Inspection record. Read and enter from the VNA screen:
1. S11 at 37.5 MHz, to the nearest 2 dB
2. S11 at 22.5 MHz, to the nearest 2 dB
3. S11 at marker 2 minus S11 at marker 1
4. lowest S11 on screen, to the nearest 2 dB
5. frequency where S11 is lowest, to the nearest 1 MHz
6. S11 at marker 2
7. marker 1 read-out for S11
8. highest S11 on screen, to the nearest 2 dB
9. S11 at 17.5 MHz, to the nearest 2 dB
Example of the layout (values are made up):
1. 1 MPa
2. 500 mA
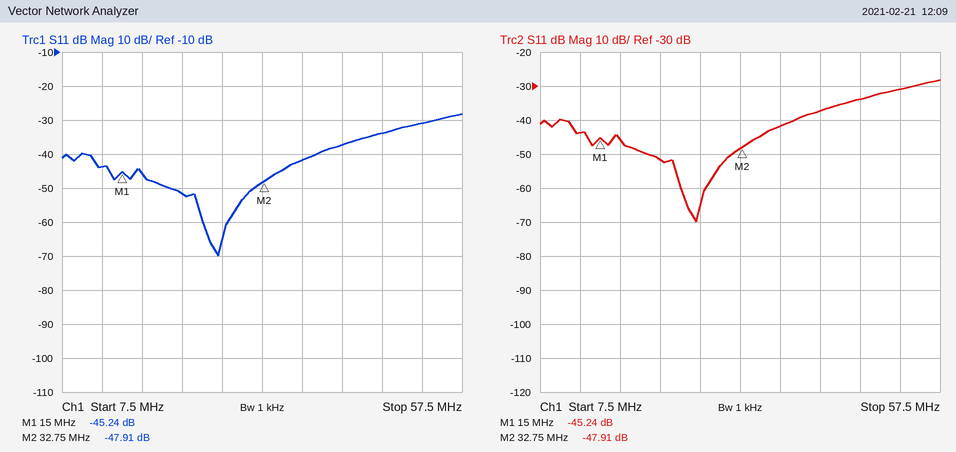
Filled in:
1. -42 dB
2. -52 dB
3. -2.67 dB
4. -70 dB
5. 27 MHz
6. -47.91 dB
7. -45.24 dB
8. -28 dB
9. -46 dB
